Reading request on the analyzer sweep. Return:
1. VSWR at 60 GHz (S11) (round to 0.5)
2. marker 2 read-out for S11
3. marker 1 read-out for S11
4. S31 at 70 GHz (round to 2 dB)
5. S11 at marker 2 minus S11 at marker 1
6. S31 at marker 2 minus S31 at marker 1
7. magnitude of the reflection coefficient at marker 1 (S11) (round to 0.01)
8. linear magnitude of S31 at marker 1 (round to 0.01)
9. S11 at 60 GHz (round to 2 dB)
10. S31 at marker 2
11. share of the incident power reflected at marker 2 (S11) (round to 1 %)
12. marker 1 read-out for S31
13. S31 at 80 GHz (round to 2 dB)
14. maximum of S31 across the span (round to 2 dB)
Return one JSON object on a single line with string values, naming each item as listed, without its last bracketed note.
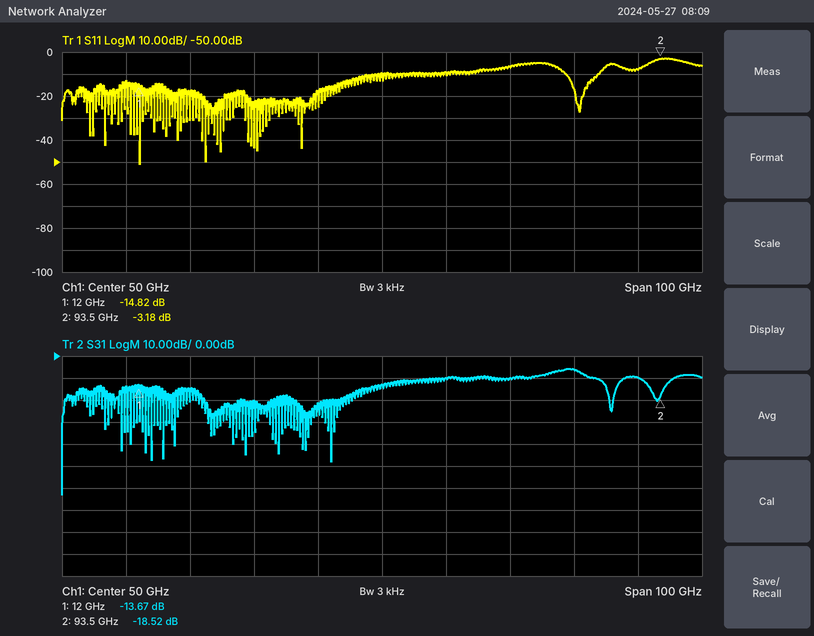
{"VSWR at 60 GHz (S11)": "2.0", "marker 2 read-out for S11": "-3.18 dB", "marker 1 read-out for S11": "-14.82 dB", "S31 at 70 GHz": "-10 dB", "S11 at marker 2 minus S11 at marker 1": "11.64 dB", "S31 at marker 2 minus S31 at marker 1": "-4.85 dB", "magnitude of the reflection coefficient at marker 1 (S11)": "0.18", "linear magnitude of S31 at marker 1": "0.21", "S11 at 60 GHz": "-10 dB", "S31 at marker 2": "-18.52 dB", "share of the incident power reflected at marker 2 (S11)": "48 %", "marker 1 read-out for S31": "-13.67 dB", "S31 at 80 GHz": "-6 dB", "maximum of S31 across the span": "-6 dB"}
